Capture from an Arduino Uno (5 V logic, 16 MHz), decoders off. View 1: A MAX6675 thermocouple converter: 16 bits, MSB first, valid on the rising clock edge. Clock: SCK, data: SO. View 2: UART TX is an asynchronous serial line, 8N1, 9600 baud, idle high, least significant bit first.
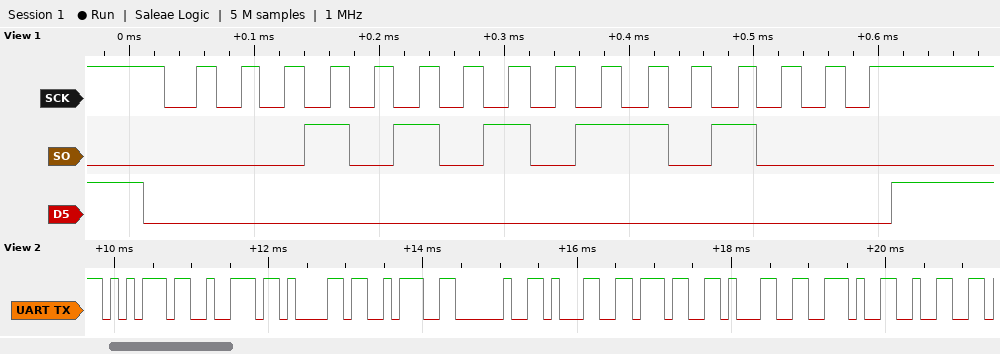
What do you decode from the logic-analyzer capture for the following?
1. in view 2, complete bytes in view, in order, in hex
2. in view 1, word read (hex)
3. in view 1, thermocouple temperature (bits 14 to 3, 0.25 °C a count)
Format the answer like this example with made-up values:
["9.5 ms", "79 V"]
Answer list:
["0x75 0x72 0x61 0x3A 0x20 0x31 0x37 0x31 0x2E 0x32", "0x1568", "171.25 °C"]
